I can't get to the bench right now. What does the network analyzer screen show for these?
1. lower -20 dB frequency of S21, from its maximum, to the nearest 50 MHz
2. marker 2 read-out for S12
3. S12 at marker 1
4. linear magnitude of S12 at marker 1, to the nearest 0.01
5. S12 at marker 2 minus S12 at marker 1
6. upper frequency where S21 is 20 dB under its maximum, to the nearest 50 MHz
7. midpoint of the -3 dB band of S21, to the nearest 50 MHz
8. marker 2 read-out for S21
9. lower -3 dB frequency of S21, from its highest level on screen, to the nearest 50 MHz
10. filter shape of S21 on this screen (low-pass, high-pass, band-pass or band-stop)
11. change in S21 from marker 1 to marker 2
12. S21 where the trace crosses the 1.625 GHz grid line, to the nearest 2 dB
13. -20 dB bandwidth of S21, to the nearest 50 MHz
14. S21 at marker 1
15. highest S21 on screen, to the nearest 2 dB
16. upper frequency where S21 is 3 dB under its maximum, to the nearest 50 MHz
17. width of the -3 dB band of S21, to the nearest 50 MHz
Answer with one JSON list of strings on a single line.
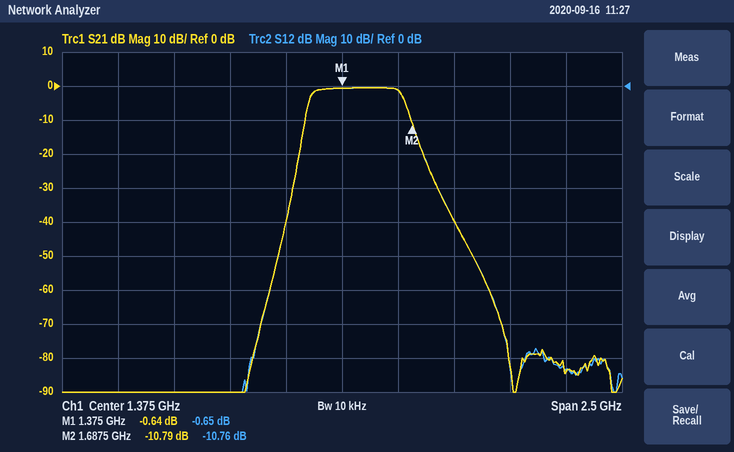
["1.20 GHz", "-10.76 dB", "-0.65 dB", "0.93", "-10.11 dB", "1.75 GHz", "1.45 GHz", "-10.79 dB", "1.25 GHz", "band-pass", "-10.15 dB", "-2 dB", "550 MHz", "-0.64 dB", "0 dB", "1.65 GHz", "400 MHz"]
